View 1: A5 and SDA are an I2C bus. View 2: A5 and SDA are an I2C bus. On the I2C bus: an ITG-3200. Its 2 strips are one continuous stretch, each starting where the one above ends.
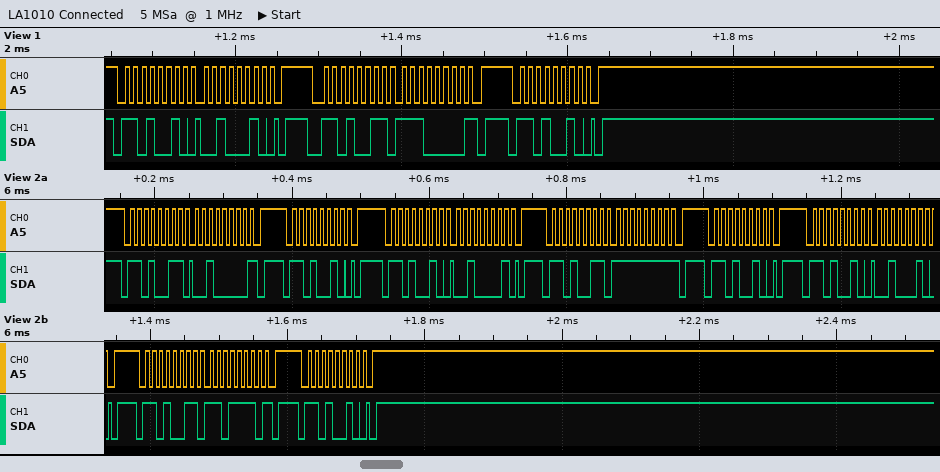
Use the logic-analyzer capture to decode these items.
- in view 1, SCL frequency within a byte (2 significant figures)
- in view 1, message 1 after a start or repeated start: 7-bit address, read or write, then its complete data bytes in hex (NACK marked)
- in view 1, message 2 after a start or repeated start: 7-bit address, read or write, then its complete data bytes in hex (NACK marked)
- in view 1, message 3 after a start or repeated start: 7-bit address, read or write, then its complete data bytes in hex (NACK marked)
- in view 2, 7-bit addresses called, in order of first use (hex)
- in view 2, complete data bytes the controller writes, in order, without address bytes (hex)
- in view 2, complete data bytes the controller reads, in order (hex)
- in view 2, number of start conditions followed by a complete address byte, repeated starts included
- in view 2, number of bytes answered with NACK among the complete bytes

100 kHz
0x69 write: 22
0x69 read: E0 NACK
0x69 write
0x69
21 22
20 FF DE
8
3
